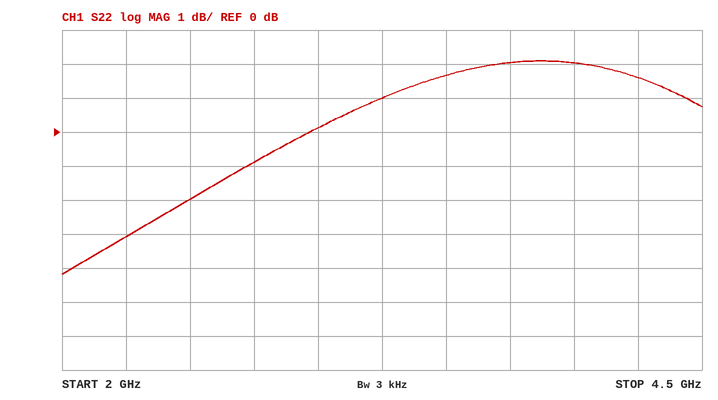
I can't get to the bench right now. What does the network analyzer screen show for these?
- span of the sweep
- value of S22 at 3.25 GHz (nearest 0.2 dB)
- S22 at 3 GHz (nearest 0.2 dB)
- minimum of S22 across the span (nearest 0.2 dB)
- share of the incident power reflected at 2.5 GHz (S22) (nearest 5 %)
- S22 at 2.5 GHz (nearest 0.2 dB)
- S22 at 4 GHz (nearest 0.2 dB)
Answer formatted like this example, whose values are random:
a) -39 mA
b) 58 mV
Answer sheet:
a) 2.5 GHz
b) 1.0 dB
c) 0.2 dB
d) -4.2 dB
e) 65 %
f) -2.0 dB
g) 2.0 dB
